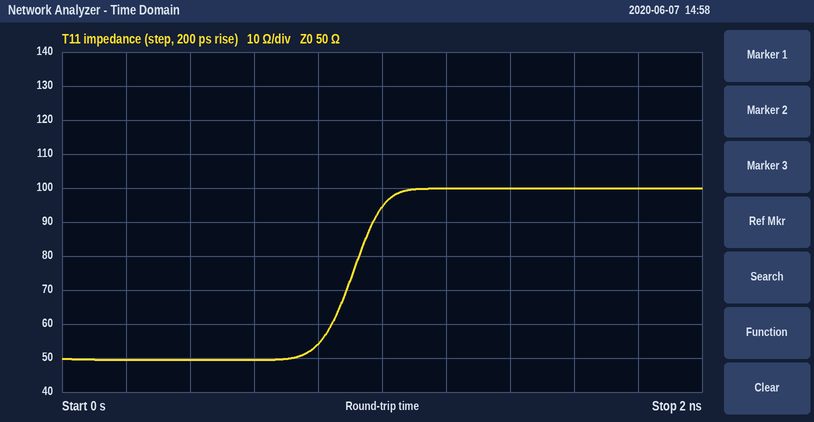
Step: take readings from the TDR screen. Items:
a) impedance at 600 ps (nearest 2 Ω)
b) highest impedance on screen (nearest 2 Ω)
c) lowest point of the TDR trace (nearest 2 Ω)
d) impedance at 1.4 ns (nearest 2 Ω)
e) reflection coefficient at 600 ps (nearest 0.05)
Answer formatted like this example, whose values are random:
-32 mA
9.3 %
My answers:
50 Ω
100 Ω
50 Ω
100 Ω
0.00
